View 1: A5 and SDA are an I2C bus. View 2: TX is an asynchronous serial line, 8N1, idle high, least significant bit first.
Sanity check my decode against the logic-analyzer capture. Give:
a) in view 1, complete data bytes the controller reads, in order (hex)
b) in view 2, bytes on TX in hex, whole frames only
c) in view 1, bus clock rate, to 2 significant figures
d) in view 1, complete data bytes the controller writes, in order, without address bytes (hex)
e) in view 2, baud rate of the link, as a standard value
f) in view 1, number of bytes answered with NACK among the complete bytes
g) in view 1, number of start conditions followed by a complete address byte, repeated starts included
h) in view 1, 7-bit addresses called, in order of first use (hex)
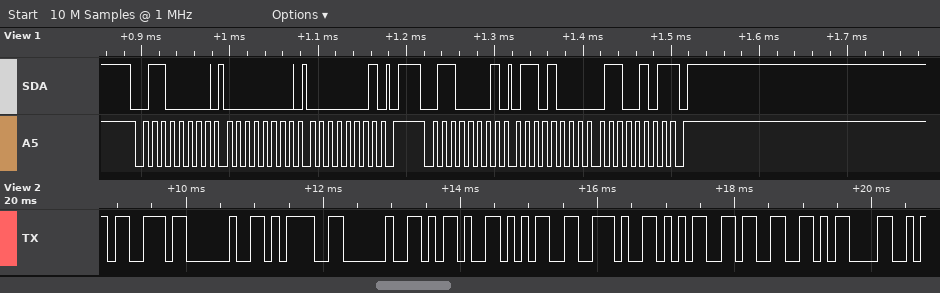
68 65
73 20 3D 20 2D 35 2E 35 33 0D
100 kHz
00 01
9600 baud
1
2
0x30
